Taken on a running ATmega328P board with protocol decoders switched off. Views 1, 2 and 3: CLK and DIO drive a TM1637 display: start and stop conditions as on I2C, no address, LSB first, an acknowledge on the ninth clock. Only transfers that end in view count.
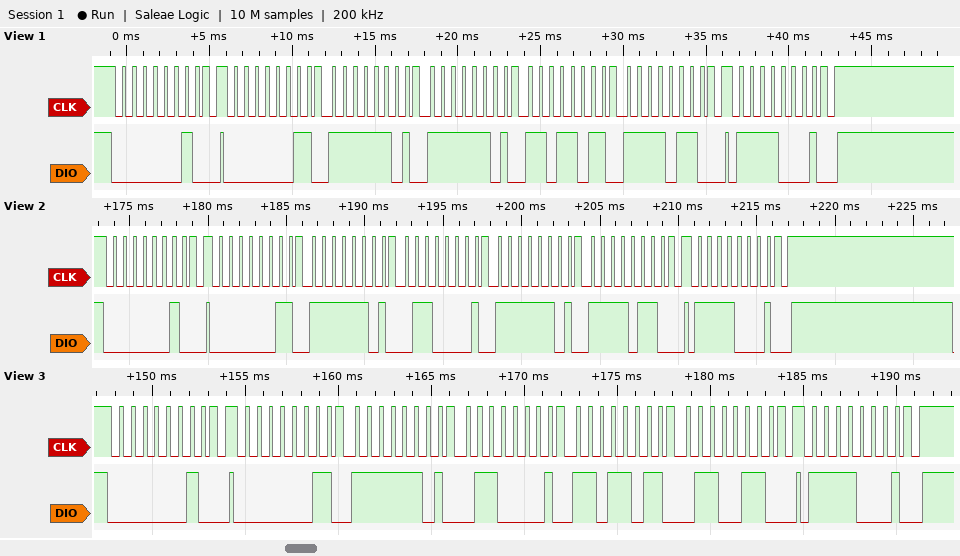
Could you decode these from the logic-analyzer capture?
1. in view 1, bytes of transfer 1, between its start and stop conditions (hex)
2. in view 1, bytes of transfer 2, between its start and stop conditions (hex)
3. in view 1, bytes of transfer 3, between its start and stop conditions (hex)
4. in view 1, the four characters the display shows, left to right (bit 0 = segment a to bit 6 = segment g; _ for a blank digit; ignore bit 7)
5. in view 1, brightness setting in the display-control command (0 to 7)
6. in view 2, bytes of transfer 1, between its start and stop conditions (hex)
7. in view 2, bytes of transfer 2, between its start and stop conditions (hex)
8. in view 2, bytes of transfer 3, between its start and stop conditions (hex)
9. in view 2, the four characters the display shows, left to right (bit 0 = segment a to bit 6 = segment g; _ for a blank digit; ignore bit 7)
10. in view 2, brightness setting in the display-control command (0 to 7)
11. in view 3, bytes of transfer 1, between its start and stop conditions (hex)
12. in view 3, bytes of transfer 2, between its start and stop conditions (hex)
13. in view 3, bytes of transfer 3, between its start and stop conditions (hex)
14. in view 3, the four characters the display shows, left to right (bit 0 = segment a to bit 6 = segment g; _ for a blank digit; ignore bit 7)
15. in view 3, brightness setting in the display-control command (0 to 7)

40
C0 BF BF DB 6F
8F
0029
7
40
C0 BF 86 BF 6F
8F
0109
7
40
C0 BF 86 DB 66
8F
0124
7
